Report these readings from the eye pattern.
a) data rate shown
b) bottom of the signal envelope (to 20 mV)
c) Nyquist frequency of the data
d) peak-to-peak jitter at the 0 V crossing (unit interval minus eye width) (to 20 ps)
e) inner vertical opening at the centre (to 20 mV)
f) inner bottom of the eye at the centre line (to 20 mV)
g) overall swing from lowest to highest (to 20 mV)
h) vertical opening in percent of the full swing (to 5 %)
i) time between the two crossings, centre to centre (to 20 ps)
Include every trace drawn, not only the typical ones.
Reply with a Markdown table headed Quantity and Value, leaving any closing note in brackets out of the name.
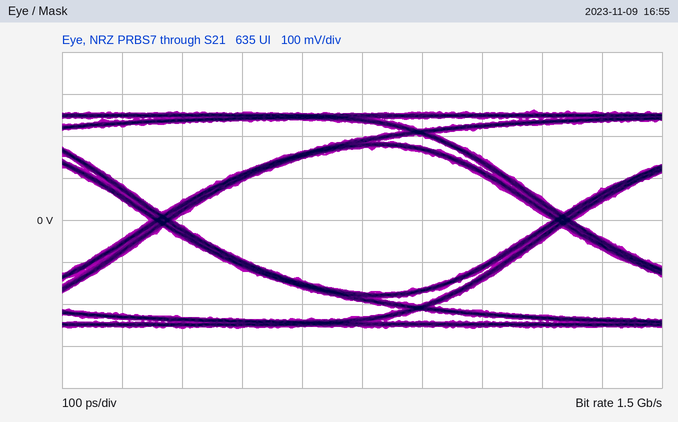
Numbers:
| Quantity | Value |
|---|---|
| data rate shown | 1.5 Gb/s |
| bottom of the signal envelope | -260 mV |
| Nyquist frequency of the data | 750 MHz |
| peak-to-peak jitter at the 0 V crossing (unit interval minus eye width) | 40 ps |
| inner vertical opening at the centre | 340 mV |
| inner bottom of the eye at the centre line | -180 mV |
| overall swing from lowest to highest | 520 mV |
| vertical opening in percent of the full swing | 65 % |
| time between the two crossings, centre to centre | 660 ps |
